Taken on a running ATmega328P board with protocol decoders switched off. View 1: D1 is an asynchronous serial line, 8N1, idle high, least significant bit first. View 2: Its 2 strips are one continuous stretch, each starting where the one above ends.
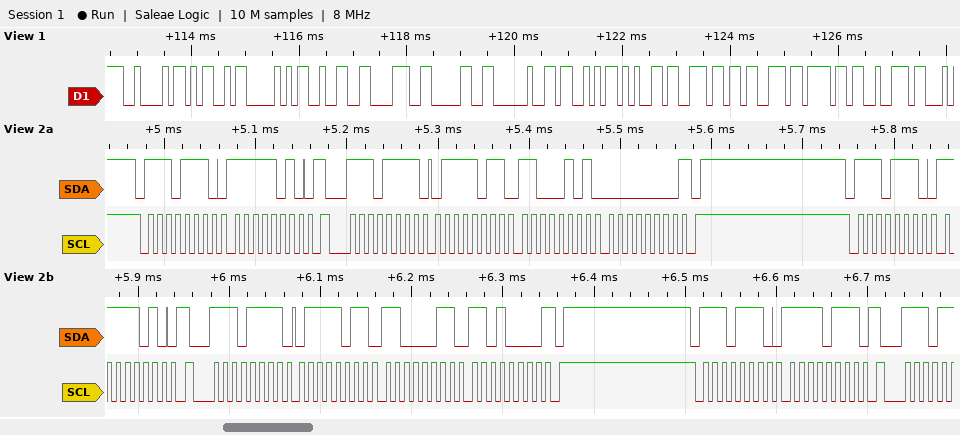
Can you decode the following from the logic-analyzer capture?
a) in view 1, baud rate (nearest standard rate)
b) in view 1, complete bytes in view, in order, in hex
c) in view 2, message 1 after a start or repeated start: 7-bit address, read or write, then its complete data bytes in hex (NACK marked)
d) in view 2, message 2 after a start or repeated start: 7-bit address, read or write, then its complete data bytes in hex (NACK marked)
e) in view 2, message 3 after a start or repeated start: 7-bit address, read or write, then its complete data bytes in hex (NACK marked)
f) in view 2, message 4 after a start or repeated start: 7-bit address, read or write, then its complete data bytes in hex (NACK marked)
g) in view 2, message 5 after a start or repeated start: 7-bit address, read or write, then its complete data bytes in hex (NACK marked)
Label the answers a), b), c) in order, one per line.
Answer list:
a) 9600 baud
b) 42 4D 50 32 38 30 20 53 65 6E 73 6F 72
c) 0x77 write: FA
d) 0x77 read: 7B C5 00 NACK
e) 0x77 write: FA
f) 0x77 read: 7B C3 D0 NACK
g) 0x77 write: F7
